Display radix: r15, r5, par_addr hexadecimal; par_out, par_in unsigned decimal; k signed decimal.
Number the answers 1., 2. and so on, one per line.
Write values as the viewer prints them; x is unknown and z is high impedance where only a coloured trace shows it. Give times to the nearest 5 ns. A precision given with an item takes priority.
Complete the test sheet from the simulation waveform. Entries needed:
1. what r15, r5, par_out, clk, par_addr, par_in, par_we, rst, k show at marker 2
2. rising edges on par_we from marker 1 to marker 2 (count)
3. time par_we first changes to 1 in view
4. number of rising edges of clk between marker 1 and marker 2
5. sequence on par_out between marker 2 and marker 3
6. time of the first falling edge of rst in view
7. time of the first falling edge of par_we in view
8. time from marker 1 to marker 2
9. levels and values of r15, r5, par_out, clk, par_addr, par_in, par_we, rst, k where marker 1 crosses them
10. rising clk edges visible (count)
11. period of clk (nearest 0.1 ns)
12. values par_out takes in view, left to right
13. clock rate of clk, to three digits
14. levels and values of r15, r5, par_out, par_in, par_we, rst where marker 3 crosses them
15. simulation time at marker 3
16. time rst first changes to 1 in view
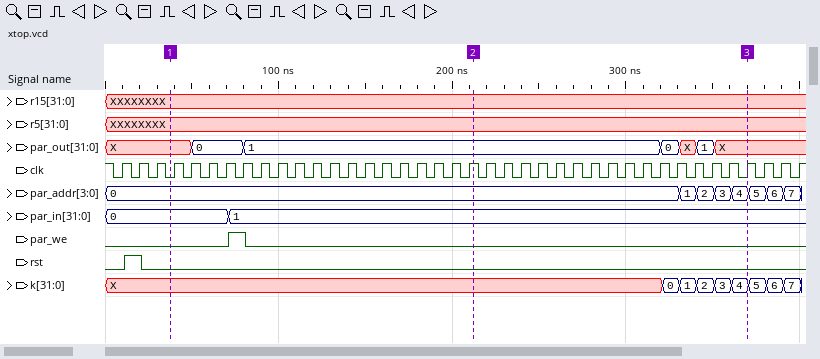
1. r15=XXXXXXXX, r5=XXXXXXXX, par_out=1, clk=1, par_addr=0, par_in=1, par_we=0, rst=0, k=X
2. 1
3. 70 ns
4. 18
5. 1, 0, X, 1, X
6. 20 ns
7. 80 ns
8. 175 ns
9. r15=XXXXXXXX, r5=XXXXXXXX, par_out=X, clk=0, par_addr=0, par_in=0, par_we=0, rst=0, k=X
10. 40
11. 10 ns
12. X, 0, 1, 0, X, 1, X
13. 100 MHz
14. r15=XXXXXXXX, r5=XXXXXXXX, par_out=X, par_in=1, par_we=0, rst=0
15. 370 ns
16. 10 ns
